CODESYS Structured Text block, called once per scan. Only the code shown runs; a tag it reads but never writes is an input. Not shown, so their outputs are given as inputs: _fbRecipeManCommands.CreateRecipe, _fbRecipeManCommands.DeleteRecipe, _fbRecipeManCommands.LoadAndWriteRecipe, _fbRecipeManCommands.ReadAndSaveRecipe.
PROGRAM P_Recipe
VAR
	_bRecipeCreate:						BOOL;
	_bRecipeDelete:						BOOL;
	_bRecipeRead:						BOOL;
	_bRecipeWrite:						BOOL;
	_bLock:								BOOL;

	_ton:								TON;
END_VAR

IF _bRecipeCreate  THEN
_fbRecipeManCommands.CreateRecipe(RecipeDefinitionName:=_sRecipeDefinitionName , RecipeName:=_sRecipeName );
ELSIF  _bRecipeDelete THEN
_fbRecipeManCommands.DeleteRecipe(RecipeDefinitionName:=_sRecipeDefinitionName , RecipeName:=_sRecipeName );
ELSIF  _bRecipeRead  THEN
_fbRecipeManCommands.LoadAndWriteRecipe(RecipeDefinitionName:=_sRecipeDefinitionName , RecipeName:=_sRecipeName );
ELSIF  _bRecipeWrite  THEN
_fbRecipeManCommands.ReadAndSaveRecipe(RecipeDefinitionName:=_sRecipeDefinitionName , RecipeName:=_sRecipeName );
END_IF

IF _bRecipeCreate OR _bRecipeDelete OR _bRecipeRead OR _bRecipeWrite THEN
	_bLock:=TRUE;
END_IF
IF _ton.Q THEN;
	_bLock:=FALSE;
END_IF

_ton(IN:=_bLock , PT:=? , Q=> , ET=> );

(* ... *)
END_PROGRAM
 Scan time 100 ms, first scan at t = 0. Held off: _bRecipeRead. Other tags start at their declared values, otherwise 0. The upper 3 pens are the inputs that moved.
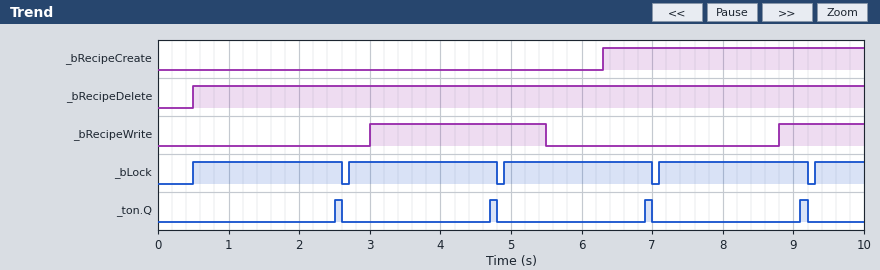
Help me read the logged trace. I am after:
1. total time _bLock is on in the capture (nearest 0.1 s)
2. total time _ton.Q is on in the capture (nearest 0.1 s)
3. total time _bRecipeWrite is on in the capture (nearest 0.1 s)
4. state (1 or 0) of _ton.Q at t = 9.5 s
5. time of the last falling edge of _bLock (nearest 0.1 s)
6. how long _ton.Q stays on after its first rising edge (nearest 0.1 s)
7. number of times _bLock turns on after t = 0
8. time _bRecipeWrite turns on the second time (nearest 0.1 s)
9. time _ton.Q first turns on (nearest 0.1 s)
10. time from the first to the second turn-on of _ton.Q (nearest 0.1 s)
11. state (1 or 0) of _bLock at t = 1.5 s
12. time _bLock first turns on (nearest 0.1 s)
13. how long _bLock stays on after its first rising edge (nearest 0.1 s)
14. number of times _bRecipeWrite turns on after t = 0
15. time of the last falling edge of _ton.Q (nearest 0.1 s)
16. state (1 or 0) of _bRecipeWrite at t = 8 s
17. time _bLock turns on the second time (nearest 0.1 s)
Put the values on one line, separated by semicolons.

9.1 s; 0.4 s; 3.7 s; 0; 9.2 s; 0.1 s; 5; 8.8 s; 2.5 s; 2.2 s; 1; 0.5 s; 2.1 s; 2; 9.2 s; 0; 2.7 s
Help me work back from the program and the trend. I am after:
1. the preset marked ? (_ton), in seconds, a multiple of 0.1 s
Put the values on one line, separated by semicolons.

2.0 s
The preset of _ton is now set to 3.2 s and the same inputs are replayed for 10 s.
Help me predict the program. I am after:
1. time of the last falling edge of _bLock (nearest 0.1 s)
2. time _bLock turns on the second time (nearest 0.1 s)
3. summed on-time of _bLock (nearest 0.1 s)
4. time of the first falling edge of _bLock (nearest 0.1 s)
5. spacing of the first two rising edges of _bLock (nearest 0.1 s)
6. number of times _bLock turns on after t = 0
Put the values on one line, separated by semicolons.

7.2 s; 3.9 s; 9.3 s; 3.8 s; 3.4 s; 3
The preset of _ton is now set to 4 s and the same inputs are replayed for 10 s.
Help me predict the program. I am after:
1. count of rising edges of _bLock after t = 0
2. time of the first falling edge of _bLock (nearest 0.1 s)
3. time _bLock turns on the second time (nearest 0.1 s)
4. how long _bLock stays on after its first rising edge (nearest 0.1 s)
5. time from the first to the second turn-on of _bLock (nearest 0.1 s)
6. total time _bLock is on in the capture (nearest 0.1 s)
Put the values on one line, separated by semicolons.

3; 4.6 s; 4.7 s; 4.1 s; 4.2 s; 9.3 s
